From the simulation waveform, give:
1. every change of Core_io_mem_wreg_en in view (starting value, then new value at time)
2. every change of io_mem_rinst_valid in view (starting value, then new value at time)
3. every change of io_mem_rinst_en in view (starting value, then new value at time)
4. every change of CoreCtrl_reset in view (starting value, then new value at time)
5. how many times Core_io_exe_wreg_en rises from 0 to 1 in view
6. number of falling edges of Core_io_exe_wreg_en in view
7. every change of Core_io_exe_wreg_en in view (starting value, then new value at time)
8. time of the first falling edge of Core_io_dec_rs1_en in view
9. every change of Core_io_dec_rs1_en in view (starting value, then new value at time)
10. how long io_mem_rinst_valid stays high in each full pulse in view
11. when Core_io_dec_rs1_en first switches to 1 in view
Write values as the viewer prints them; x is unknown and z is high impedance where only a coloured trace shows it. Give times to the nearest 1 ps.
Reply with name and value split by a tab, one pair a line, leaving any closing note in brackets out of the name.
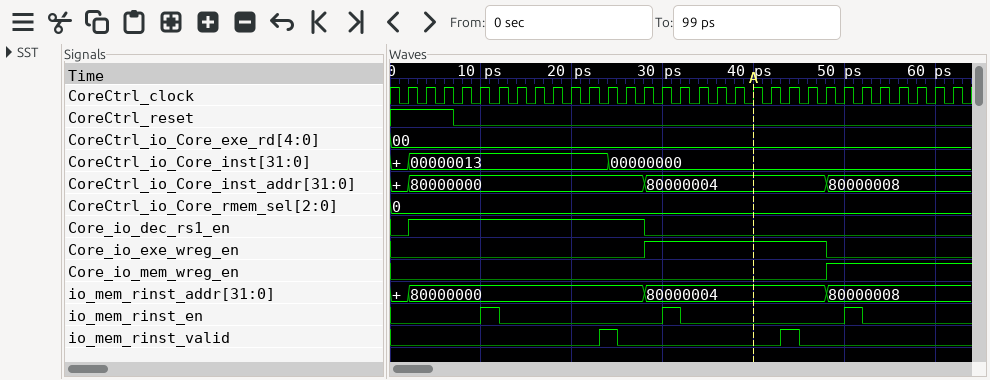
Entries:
every change of Core_io_mem_wreg_en in view	0, 1 at 48 ps
every change of io_mem_rinst_valid in view	0, 1 at 23 ps, 0 at 25 ps, 1 at 43 ps, 0 at 45 ps
every change of io_mem_rinst_en in view	0, 1 at 10 ps, 0 at 12 ps, 1 at 30 ps, 0 at 32 ps, 1 at 50 ps, 0 at 52 ps
every change of CoreCtrl_reset in view	1, 0 at 7 ps
how many times Core_io_exe_wreg_en rises from 0 to 1 in view	1
number of falling edges of Core_io_exe_wreg_en in view	1
every change of Core_io_exe_wreg_en in view	0, 1 at 28 ps, 0 at 48 ps
time of the first falling edge of Core_io_dec_rs1_en in view	28 ps
every change of Core_io_dec_rs1_en in view	0, 1 at 2 ps, 0 at 28 ps
how long io_mem_rinst_valid stays high in each full pulse in view	2 ps, 2 ps
when Core_io_dec_rs1_en first switches to 1 in view	2 ps
